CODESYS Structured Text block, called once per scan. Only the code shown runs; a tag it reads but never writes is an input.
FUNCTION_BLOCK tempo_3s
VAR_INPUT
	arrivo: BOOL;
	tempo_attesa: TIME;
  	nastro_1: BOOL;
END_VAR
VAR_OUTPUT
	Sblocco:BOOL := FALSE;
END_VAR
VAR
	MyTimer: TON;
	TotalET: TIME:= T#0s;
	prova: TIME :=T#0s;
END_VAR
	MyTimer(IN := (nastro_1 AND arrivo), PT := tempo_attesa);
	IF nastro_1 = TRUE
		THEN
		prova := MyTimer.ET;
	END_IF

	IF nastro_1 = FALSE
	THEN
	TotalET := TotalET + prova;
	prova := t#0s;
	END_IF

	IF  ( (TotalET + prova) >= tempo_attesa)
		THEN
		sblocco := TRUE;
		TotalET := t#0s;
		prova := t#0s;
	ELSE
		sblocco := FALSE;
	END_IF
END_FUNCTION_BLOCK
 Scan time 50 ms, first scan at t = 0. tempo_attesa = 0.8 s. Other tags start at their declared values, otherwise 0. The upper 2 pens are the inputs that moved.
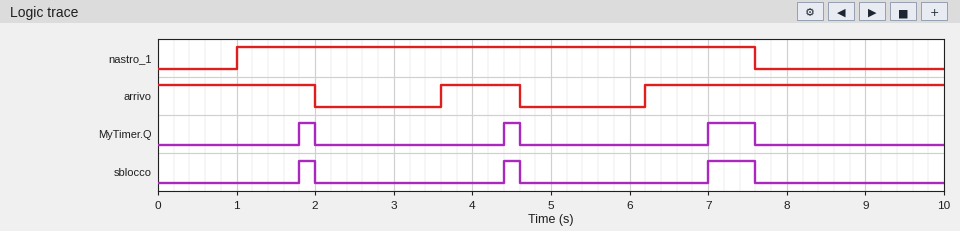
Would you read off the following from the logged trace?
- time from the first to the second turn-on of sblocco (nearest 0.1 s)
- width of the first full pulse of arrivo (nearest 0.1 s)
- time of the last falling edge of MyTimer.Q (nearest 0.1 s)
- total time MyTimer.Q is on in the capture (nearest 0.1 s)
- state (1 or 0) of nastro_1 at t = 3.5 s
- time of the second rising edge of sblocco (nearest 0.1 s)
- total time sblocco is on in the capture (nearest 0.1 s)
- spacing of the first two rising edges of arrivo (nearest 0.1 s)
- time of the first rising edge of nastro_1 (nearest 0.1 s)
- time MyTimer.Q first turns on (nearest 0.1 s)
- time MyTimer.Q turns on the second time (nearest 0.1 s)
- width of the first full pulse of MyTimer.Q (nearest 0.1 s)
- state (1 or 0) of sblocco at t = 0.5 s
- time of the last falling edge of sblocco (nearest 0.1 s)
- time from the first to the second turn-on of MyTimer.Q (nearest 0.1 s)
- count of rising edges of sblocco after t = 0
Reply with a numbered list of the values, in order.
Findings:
1. 2.6 s
2. 1.0 s
3. 7.6 s
4. 1.0 s
5. 1
6. 4.4 s
7. 1.0 s
8. 2.6 s
9. 1.0 s
10. 1.8 s
11. 4.4 s
12. 0.2 s
13. 0
14. 7.6 s
15. 2.6 s
16. 3
